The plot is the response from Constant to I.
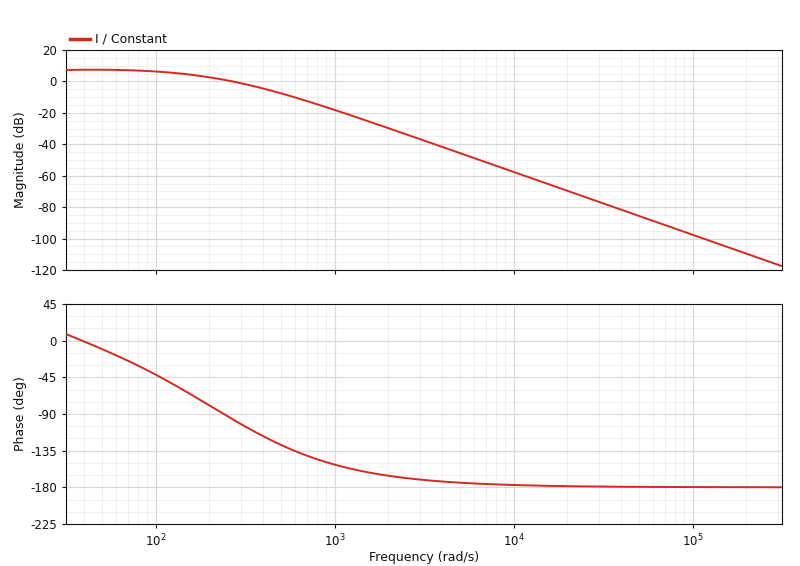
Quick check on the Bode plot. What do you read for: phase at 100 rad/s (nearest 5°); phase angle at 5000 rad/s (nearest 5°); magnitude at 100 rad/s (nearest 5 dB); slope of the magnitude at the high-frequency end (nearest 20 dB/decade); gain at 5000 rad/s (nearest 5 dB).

-40°
-175°
5 dB
-40 dB/decade
-45 dB
